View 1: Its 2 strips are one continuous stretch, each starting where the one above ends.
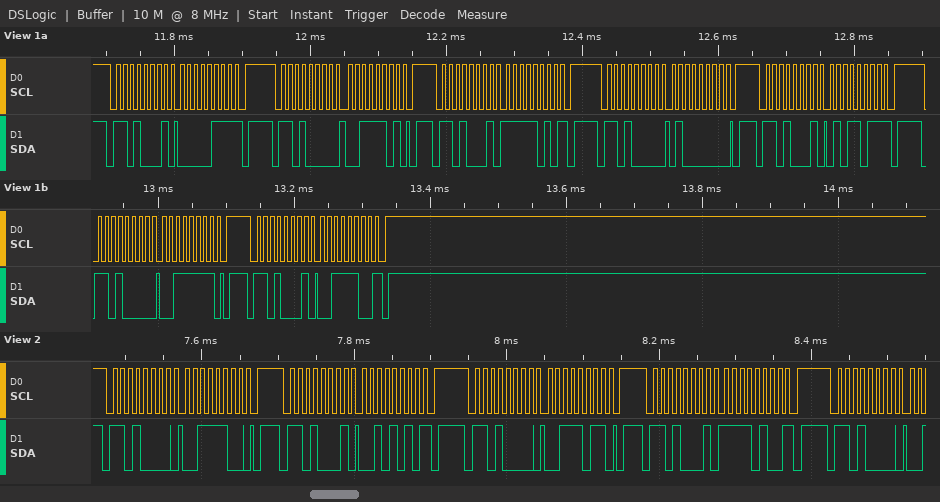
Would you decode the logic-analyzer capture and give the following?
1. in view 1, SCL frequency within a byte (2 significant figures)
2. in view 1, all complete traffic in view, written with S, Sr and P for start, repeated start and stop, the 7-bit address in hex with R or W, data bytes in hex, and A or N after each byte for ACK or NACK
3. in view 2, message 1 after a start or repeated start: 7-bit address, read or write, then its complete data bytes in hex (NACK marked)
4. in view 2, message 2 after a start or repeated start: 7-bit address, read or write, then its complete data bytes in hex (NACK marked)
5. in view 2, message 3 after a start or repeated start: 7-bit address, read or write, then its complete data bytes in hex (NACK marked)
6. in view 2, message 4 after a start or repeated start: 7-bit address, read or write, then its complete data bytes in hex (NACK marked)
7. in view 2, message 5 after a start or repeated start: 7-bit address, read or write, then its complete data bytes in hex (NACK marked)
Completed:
100 kHz
S 68R A 07 N P S 68W A 3D A P S 68R A FA N P S 68W A 40 A P S 68R A 5B N P S 68W A 3F A P S 68R A 3C N P
0x68 write: 3C
0x68 read: 2A NACK
0x68 write: 3B
0x68 read: F4 NACK
0x68 write
